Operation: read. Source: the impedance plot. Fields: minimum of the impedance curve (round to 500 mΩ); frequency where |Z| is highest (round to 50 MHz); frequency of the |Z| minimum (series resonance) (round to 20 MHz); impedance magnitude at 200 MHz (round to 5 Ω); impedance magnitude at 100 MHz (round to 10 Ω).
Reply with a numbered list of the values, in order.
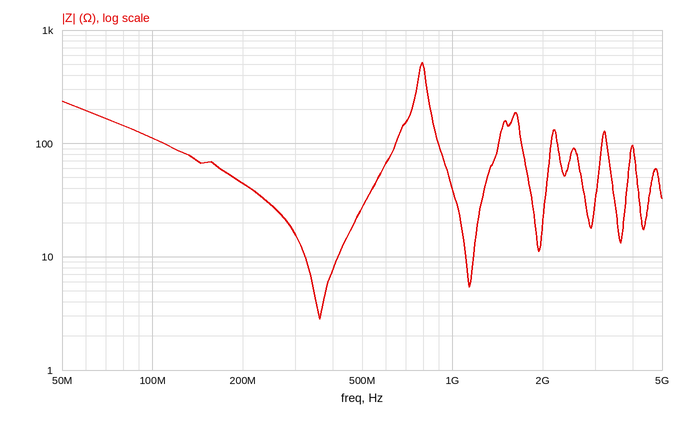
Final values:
1. 3.0 Ω
2. 800 MHz
3. 360 MHz
4. 45 Ω
5. 110 Ω
